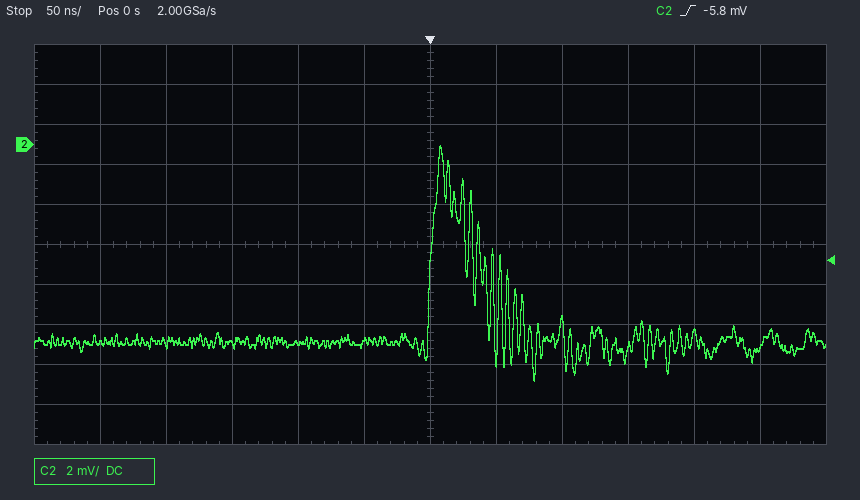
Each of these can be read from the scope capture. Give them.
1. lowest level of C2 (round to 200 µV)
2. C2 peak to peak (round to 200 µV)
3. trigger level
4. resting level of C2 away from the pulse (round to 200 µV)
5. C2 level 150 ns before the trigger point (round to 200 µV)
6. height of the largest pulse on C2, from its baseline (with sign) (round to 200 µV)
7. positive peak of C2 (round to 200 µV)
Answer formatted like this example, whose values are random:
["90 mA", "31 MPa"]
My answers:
["-11.8 mV", "11.8 mV", "-5.8 mV", "-9.8 mV", "-10.0 mV", "+9.8 mV", "0.0 mV"]
